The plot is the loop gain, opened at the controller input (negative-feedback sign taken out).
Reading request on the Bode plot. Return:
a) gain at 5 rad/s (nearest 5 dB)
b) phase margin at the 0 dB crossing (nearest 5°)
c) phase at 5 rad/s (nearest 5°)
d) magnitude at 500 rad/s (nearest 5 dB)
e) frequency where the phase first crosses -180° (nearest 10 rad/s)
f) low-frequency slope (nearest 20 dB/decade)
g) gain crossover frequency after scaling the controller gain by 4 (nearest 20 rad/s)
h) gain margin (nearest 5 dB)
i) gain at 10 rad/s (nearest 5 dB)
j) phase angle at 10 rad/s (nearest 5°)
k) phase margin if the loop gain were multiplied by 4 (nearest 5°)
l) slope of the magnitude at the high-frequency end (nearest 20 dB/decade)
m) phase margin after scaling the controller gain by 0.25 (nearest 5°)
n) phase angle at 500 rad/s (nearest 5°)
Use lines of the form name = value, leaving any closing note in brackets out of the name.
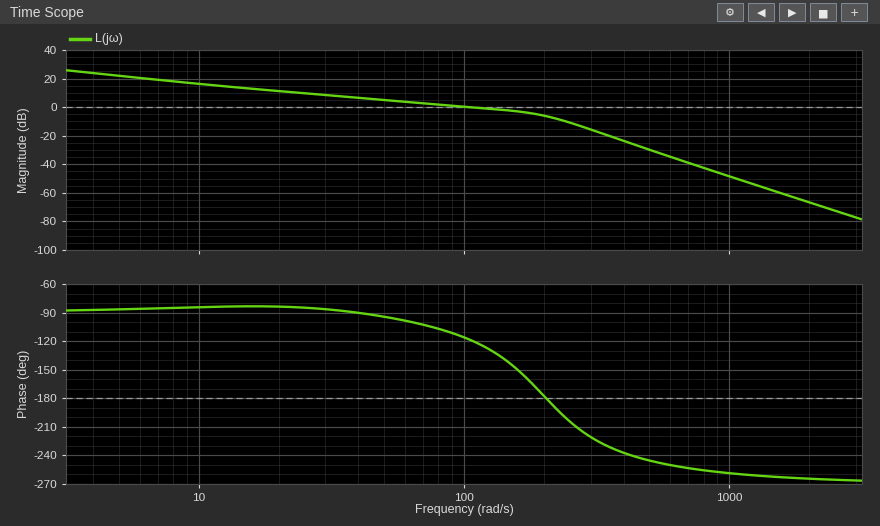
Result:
gain at 5 rad/s = 20 dB
phase margin at the 0 dB crossing = 60°
phase at 5 rad/s = -85°
magnitude at 500 rad/s = -30 dB
frequency where the phase first crosses -180° = 200 rad/s
low-frequency slope = -20 dB/decade
gain crossover frequency after scaling the controller gain by 4 = 260 rad/s
gain margin = 5 dB
gain at 10 rad/s = 15 dB
phase angle at 10 rad/s = -85°
phase margin if the loop gain were multiplied by 4 = -30°
slope of the magnitude at the high-frequency end = -60 dB/decade
phase margin after scaling the controller gain by 0.25 = 95°
phase angle at 500 rad/s = -245°
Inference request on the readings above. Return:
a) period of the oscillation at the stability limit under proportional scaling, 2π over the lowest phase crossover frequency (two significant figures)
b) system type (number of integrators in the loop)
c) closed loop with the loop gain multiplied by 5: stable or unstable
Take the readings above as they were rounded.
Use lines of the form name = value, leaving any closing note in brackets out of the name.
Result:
period of the oscillation at the stability limit under proportional scaling, 2π over the lowest phase crossover frequency = 0.031 s
system type = 1
closed loop with the loop gain multiplied by 5: stable or unstable = unstable
